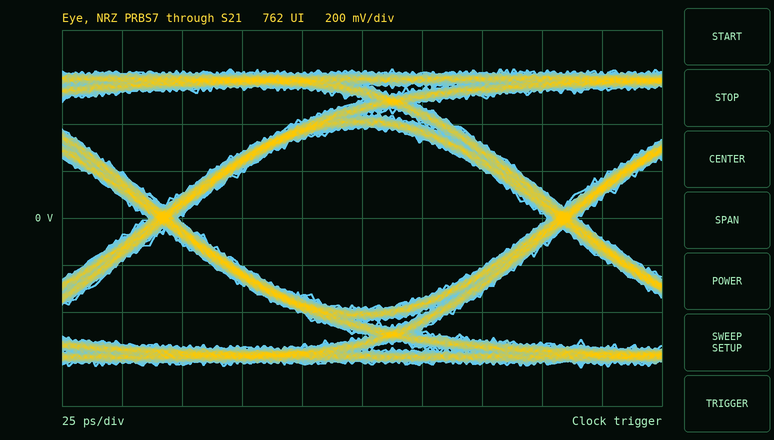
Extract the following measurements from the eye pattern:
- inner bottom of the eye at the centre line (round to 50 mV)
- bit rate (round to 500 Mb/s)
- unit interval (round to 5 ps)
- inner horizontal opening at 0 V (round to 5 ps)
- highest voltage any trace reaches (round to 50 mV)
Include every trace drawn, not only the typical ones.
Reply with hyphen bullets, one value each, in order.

- -400 mV
- 6.0 Gb/s
- 165 ps
- 155 ps
- 650 mV
